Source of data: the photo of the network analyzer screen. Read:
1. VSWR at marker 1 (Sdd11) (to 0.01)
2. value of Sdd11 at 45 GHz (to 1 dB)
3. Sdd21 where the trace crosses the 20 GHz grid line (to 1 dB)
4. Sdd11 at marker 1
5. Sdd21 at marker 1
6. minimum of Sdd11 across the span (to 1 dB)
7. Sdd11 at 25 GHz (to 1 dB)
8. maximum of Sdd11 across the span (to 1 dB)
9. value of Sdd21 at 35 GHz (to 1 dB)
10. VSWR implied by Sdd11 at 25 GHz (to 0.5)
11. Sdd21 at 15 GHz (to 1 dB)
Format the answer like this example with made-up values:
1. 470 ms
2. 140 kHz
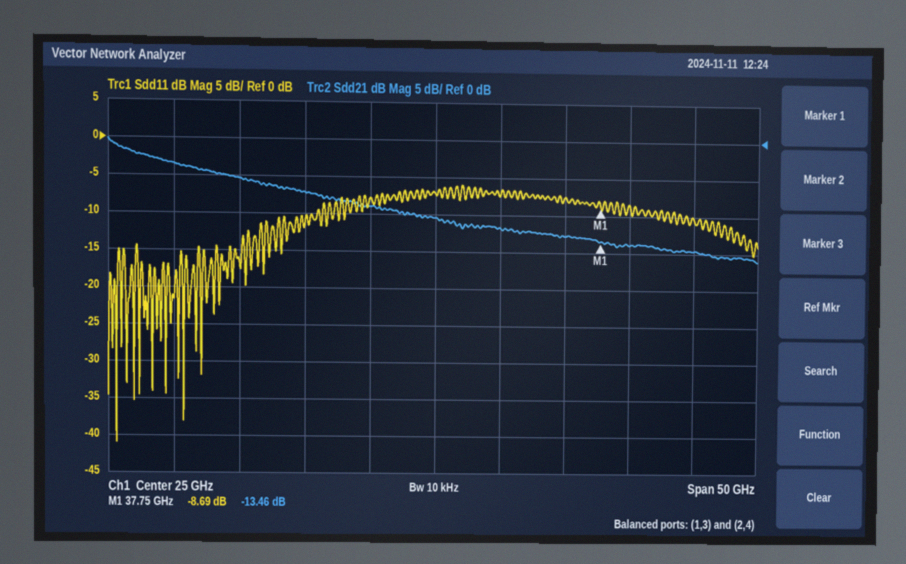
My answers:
1. 2.16
2. -10 dB
3. -9 dB
4. -8.69 dB
5. -13.46 dB
6. -41 dB
7. -7 dB
8. -6 dB
9. -13 dB
10. 2.5
11. -7 dB
